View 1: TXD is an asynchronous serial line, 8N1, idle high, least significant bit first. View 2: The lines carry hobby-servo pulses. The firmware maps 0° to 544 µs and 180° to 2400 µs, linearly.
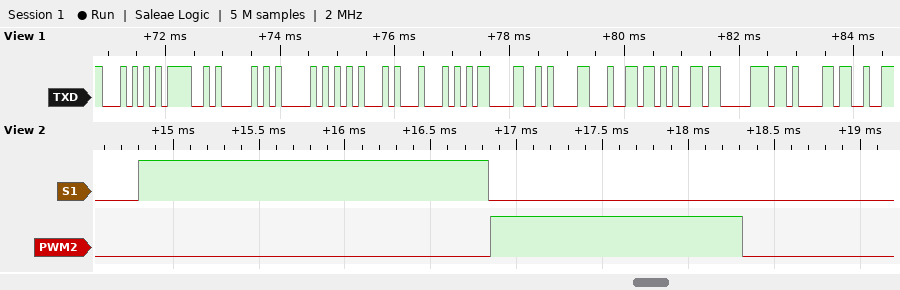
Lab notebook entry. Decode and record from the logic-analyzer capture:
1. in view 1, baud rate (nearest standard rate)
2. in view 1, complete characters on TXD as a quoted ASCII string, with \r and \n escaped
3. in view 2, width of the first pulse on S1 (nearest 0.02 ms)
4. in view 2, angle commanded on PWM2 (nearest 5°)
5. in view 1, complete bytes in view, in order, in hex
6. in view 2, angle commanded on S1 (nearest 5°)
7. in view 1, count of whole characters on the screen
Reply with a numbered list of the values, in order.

1. 9600 baud
2. "TOPPED\r\ndepa"
3. 2.04 ms
4. 90°
5. 54 4F 50 50 45 44 0D 0A 64 65 70 61
6. 145°
7. 12
